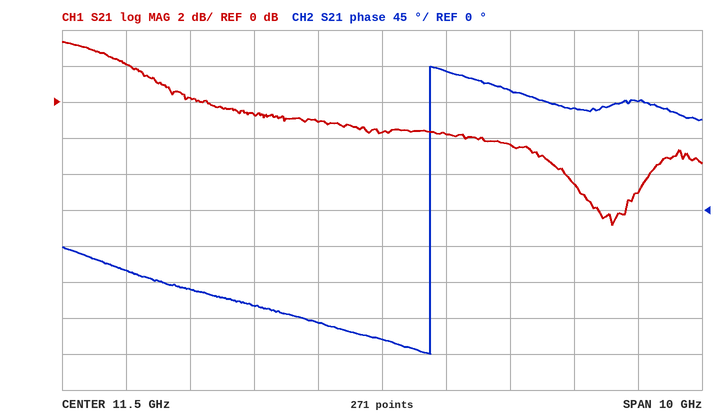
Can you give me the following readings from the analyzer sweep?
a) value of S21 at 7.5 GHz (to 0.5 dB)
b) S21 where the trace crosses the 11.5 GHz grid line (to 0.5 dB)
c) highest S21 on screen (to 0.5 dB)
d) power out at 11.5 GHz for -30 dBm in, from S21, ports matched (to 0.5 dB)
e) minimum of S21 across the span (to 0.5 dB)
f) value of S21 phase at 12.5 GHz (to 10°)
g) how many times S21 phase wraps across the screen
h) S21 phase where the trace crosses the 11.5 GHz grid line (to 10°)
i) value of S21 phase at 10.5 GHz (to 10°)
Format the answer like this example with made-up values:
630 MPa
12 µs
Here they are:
2.0 dB
-1.5 dB
3.5 dB
-31.5 dBm
-7.0 dB
170°
1
-160°
-140°
